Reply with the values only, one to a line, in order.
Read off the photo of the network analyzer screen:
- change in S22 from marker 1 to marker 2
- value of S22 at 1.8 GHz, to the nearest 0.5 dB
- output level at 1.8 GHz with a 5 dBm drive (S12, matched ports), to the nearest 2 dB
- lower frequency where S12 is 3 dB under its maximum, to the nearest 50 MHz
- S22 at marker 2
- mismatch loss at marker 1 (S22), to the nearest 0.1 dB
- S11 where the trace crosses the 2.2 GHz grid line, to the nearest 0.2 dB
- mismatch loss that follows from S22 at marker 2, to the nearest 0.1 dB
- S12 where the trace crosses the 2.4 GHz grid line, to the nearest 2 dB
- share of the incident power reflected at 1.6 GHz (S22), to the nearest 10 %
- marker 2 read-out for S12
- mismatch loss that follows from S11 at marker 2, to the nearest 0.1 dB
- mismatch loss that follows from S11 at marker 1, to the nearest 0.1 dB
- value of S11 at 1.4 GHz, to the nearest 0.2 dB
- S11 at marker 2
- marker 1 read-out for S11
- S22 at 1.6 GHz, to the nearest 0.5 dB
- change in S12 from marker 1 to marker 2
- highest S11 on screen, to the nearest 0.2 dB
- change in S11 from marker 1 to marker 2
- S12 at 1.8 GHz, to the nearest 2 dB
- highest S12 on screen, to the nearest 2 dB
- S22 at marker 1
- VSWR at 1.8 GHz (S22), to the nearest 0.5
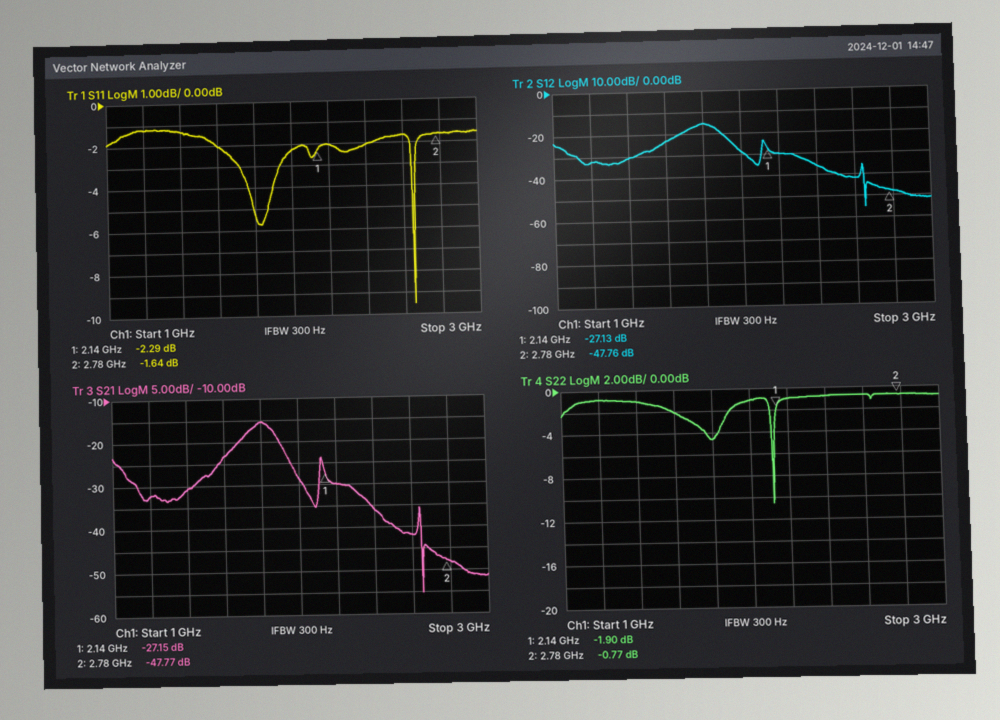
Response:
1.13 dB
-4.5 dB
-10 dBm
1.70 GHz
-0.77 dB
4.5 dB
-2.0 dB
7.9 dB
-36 dB
60 %
-47.76 dB
5.0 dB
3.9 dB
-1.4 dB
-1.64 dB
-2.29 dB
-2.0 dB
-20.63 dB
-1.2 dB
0.65 dB
-16 dB
-16 dB
-1.90 dB
4.0
